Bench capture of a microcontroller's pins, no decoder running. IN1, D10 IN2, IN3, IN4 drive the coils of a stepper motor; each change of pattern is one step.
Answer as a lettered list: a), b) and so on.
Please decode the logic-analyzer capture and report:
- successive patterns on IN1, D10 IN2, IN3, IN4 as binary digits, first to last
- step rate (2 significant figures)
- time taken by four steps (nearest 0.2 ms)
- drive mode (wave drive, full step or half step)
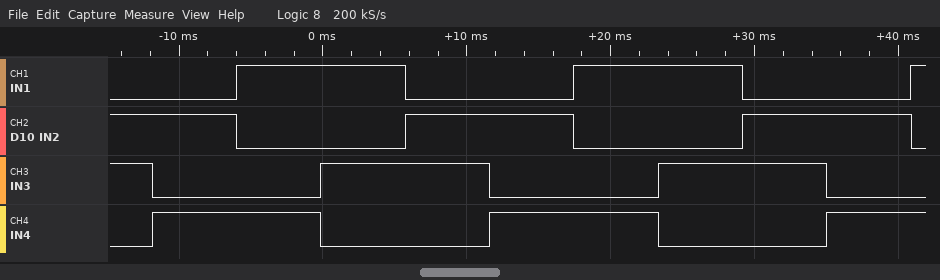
a) 0110 0101 1001 1010 0110 0101 1001 1010 0110 0101 1001
b) 170 steps/s
c) 23.4 ms
d) full step
